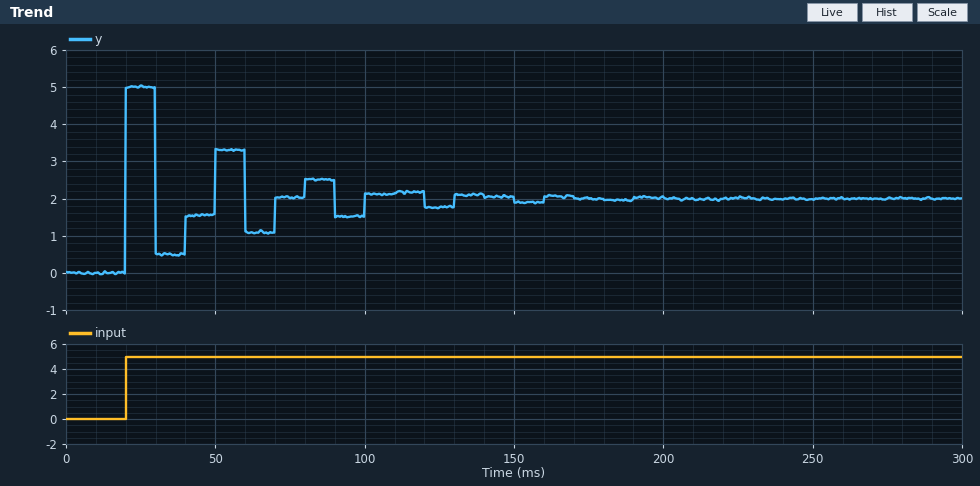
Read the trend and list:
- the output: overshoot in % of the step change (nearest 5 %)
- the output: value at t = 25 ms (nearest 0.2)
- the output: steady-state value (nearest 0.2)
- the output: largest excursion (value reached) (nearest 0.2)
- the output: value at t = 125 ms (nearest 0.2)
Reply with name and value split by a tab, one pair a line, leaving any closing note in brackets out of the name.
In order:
the output: overshoot in % of the step change	150 %
the output: value at t = 25 ms	5.0
the output: steady-state value	2.0
the output: largest excursion (value reached)	5.0
the output: value at t = 125 ms	1.8
